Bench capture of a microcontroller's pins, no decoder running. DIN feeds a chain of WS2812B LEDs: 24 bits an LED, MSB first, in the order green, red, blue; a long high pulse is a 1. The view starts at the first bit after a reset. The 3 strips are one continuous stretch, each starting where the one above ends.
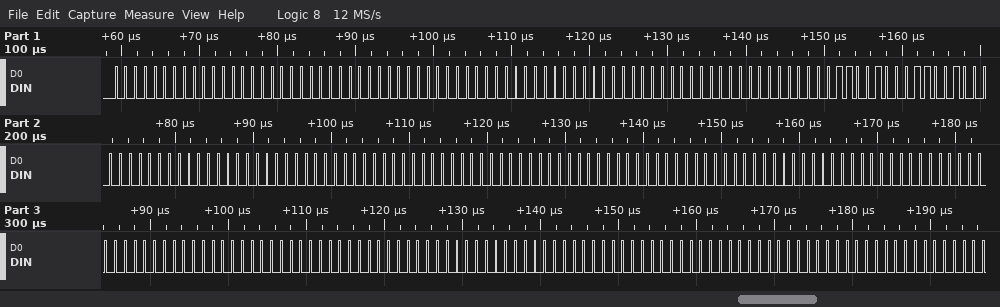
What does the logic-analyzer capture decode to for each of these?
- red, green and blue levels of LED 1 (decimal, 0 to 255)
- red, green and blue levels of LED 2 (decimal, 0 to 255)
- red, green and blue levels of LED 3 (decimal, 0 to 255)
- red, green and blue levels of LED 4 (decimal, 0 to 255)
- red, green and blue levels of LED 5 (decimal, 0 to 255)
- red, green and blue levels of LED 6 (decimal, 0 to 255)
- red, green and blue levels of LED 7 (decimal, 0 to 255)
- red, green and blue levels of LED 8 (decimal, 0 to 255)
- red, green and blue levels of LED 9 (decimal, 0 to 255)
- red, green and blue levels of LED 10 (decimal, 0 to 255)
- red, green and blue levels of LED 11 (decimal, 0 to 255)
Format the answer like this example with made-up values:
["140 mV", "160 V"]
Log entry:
["0, 0, 0", "0, 0, 0", "0, 0, 0", "50, 50, 0", "0, 0, 0", "0, 0, 0", "0, 0, 0", "0, 0, 0", "0, 0, 0", "0, 0, 0", "0, 0, 0"]
